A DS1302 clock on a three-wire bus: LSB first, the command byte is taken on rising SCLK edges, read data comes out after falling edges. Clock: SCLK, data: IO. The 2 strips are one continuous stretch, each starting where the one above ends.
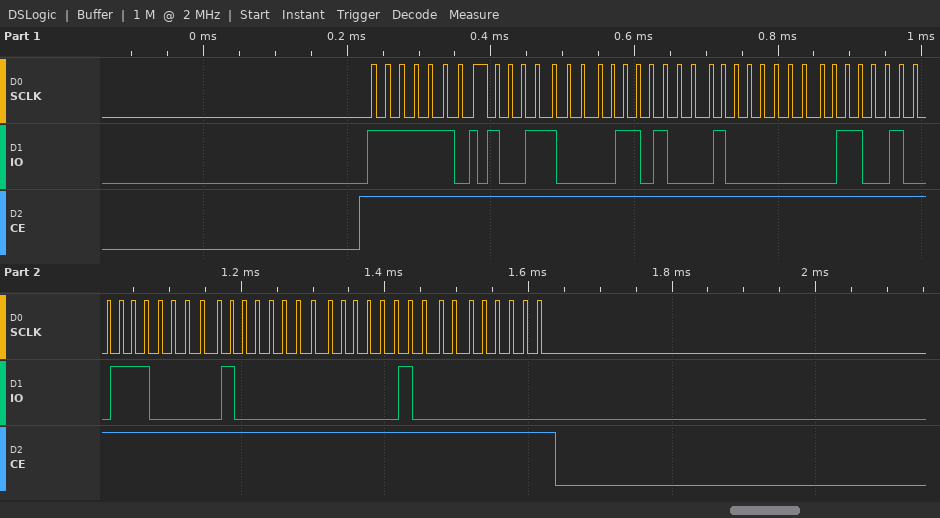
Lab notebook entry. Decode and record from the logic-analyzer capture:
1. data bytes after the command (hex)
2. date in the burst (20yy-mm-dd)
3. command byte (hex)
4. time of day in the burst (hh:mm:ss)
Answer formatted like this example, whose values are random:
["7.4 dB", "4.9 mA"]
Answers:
["19 16 01 26 07 01 20 00", "2020-07-26", "0xBF", "01:16:19"]
